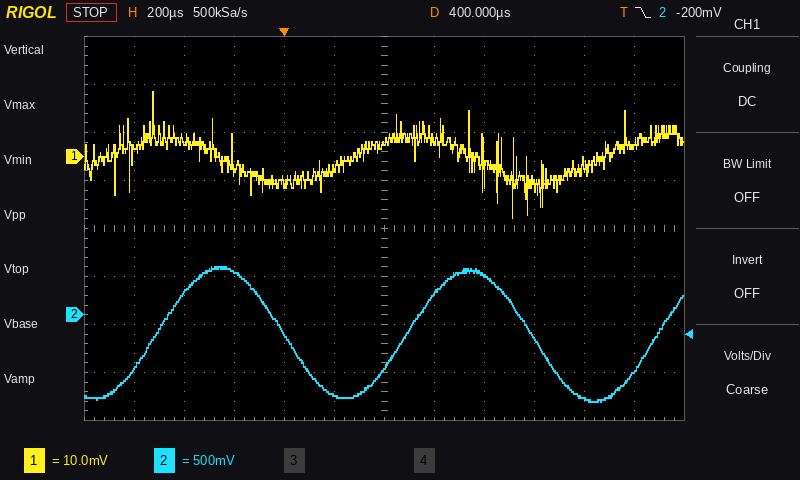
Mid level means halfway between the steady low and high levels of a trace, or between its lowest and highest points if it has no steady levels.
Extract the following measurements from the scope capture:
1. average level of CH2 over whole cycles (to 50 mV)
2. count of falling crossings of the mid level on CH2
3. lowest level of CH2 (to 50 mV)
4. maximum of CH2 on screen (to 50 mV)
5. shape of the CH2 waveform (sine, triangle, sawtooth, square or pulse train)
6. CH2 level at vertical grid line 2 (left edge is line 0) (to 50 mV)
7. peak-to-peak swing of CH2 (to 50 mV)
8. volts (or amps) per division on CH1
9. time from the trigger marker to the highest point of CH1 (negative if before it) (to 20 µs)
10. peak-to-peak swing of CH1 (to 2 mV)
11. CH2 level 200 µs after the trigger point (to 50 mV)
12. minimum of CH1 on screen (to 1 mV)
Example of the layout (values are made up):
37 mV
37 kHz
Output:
-200 mV
2
-900 mV
500 mV
sine
250 mV
1.40 V
10 mV
-520 µs
26 mV
-850 mV
-13 mV
